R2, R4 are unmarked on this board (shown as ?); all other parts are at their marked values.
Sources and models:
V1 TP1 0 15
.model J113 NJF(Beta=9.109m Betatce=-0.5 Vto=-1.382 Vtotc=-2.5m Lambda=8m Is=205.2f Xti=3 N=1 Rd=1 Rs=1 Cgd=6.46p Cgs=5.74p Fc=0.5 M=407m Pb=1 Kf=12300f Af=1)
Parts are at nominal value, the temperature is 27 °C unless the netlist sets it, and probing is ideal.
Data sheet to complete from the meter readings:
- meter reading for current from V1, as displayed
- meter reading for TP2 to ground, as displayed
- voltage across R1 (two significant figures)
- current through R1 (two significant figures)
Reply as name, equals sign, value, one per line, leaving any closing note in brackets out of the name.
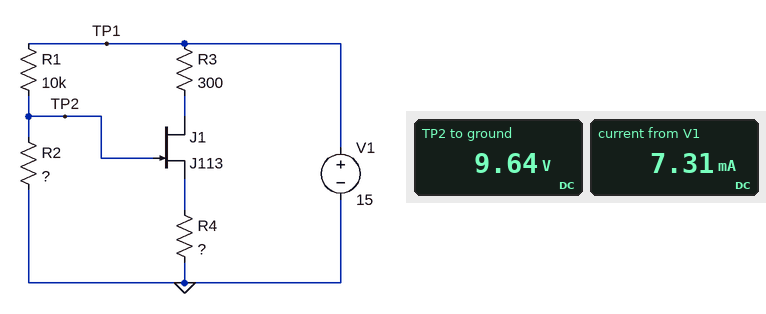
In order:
meter reading for current from V1, as displayed = 7.31 mA
meter reading for TP2 to ground, as displayed = 9.64 V
voltage across R1 = 5.4 V
current through R1 = 540 µA
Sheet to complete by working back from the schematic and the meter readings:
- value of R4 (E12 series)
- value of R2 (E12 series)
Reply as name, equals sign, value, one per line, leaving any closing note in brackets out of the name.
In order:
value of R4 = 1.5 kΩ
value of R2 = 18 kΩ
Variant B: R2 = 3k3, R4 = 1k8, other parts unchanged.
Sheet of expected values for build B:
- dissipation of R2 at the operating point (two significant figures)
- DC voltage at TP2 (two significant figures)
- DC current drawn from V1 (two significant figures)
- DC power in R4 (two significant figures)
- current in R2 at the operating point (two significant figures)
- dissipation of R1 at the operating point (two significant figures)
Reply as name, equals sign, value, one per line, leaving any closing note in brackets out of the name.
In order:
dissipation of R2 at the operating point = 4.2 mW
DC voltage at TP2 = 3.7 V
DC current drawn from V1 = 3.7 mA
DC power in R4 = 12 mW
current in R2 at the operating point = 1.1 mA
dissipation of R1 at the operating point = 13 mW
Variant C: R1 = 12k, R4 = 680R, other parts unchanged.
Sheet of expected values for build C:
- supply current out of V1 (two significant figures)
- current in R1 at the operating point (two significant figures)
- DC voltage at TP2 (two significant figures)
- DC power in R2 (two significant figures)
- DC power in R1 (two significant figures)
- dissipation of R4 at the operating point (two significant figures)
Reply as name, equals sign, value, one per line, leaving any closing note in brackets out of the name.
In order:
supply current out of V1 = 14 mA
current in R1 at the operating point = 500 µA
DC voltage at TP2 = 9.0 V
DC power in R2 = 4.5 mW
DC power in R1 = 3.0 mW
dissipation of R4 at the operating point = 120 mW
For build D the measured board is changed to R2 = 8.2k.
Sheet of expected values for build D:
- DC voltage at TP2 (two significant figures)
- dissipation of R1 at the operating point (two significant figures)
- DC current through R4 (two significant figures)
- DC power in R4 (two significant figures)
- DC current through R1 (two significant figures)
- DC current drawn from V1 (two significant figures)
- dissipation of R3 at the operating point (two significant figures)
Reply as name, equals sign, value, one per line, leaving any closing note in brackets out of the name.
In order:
DC voltage at TP2 = 6.8 V
dissipation of R1 at the operating point = 6.8 mW
DC current through R4 = 4.9 mA
DC power in R4 = 37 mW
DC current through R1 = 820 µA
DC current drawn from V1 = 5.8 mA
dissipation of R3 at the operating point = 7.3 mW
